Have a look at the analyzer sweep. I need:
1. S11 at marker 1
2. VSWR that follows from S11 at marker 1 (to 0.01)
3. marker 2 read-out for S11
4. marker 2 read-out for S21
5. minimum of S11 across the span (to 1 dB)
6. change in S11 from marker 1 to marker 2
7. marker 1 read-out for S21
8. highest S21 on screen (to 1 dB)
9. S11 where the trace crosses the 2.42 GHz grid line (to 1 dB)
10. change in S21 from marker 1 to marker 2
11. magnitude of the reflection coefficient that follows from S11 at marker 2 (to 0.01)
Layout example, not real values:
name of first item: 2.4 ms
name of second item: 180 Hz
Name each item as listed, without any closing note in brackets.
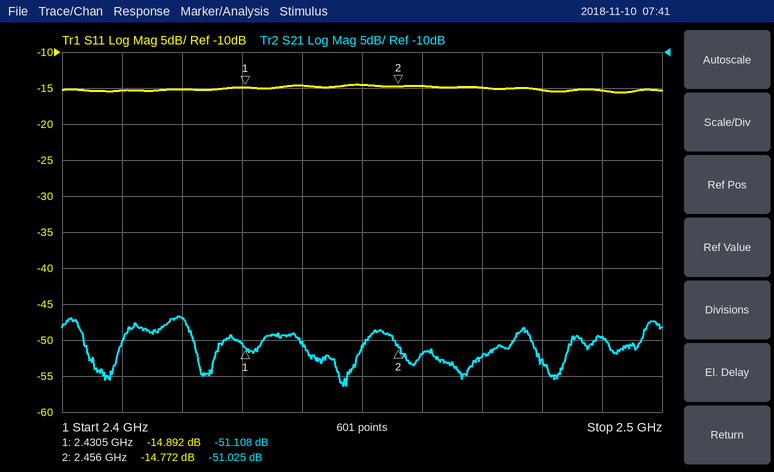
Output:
S11 at marker 1: -14.892 dB
VSWR that follows from S11 at marker 1: 1.44
marker 2 read-out for S11: -14.772 dB
marker 2 read-out for S21: -51.025 dB
minimum of S11 across the span: -16 dB
change in S11 from marker 1 to marker 2: 0.120 dB
marker 1 read-out for S21: -51.108 dB
highest S21 on screen: -47 dB
S11 where the trace crosses the 2.42 GHz grid line: -15 dB
change in S21 from marker 1 to marker 2: 0.083 dB
magnitude of the reflection coefficient that follows from S11 at marker 2: 0.18
